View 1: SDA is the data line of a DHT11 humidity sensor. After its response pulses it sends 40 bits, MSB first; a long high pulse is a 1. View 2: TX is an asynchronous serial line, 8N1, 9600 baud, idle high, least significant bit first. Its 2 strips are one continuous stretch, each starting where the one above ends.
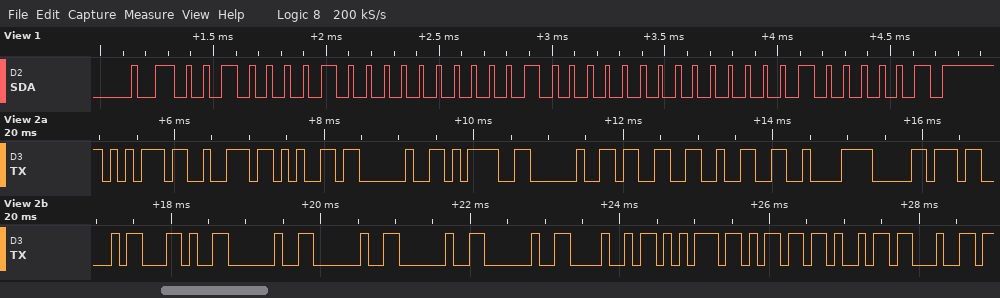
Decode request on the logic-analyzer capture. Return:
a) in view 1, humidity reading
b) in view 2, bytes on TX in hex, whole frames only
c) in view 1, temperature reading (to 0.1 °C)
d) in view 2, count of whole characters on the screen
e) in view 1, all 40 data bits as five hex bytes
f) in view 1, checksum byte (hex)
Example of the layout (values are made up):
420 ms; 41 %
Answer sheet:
33 %; 75 72 65 20 3D 20 33 32 C2 B0 43 2C 20 20 20 20 48 75 6D 69 64; 32.0 °C; 21; 21 00 20 00 41; 0x41
